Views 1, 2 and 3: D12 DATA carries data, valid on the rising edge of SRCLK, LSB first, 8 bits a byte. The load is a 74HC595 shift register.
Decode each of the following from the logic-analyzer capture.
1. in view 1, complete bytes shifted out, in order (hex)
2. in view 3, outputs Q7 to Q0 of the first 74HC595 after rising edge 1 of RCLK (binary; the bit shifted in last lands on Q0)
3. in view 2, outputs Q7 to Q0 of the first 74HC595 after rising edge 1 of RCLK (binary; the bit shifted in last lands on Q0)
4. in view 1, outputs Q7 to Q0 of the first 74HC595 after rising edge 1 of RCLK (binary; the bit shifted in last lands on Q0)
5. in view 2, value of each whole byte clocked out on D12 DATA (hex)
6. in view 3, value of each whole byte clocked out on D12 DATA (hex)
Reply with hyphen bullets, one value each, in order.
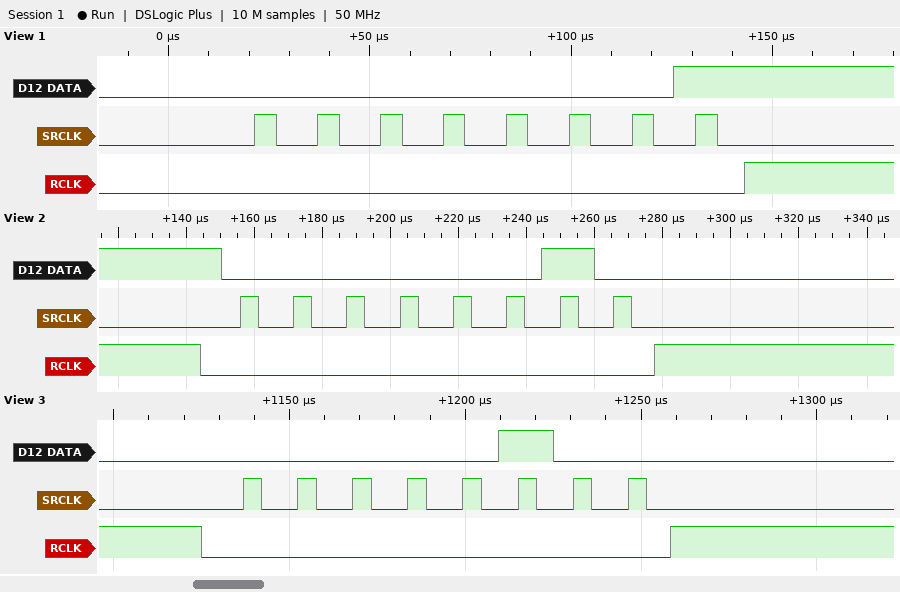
- 0x80
- 00000100
- 00000010
- 00000001
- 40
- 20
